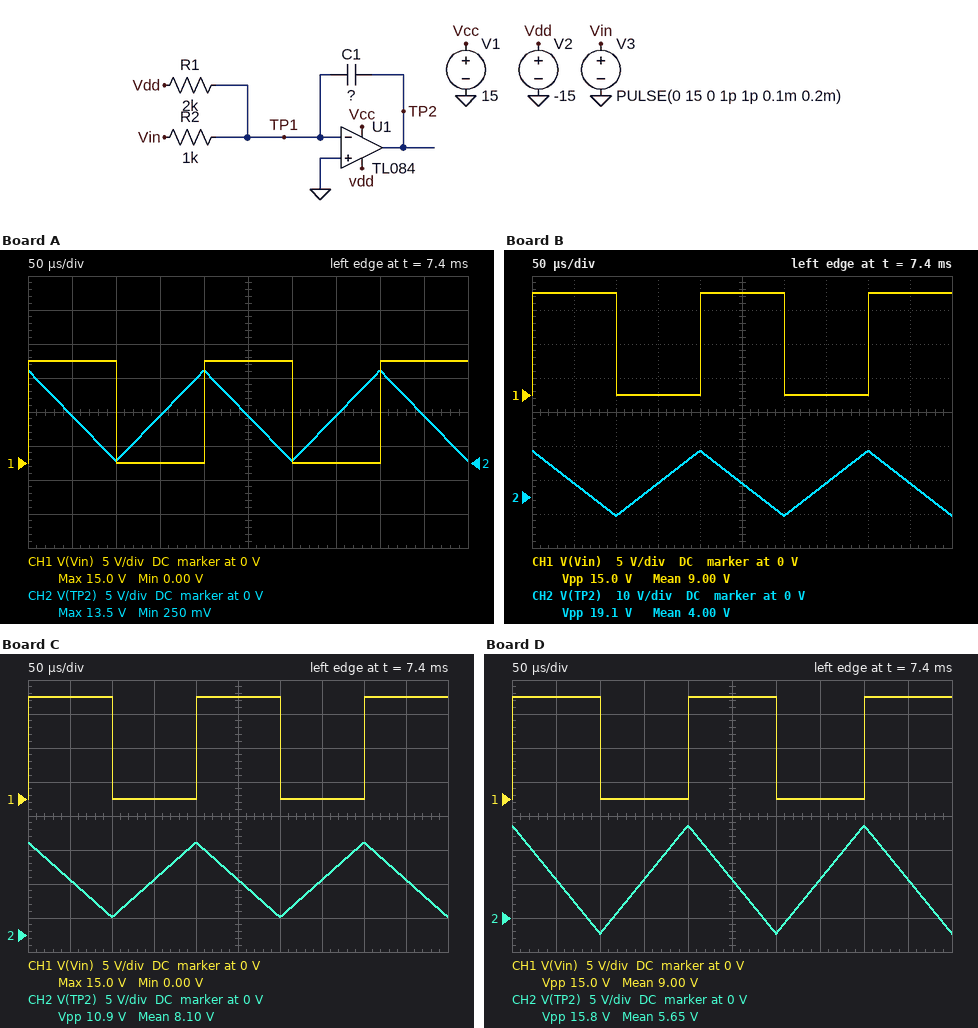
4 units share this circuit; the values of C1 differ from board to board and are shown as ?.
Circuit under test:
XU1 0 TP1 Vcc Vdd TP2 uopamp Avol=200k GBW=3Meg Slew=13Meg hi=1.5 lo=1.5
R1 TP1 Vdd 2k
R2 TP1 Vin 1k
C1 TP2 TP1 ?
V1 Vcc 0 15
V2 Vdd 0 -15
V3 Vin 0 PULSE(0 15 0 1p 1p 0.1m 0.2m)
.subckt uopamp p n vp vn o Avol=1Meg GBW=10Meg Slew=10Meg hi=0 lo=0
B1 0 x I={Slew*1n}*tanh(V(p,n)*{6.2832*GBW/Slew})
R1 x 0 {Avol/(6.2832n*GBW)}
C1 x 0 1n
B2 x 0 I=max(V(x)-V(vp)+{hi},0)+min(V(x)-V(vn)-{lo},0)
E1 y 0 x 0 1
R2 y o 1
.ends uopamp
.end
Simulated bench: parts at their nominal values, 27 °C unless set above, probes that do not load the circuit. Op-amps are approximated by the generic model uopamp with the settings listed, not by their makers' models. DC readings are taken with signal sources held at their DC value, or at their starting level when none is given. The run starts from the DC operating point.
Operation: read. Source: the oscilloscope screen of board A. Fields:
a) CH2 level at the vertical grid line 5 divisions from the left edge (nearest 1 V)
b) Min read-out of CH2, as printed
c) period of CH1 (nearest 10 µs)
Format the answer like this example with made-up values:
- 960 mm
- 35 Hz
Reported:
- 7 V
- 250 mV
- 200 µs
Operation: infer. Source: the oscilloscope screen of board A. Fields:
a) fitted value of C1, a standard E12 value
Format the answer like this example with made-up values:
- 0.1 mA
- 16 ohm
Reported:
- 56 nF
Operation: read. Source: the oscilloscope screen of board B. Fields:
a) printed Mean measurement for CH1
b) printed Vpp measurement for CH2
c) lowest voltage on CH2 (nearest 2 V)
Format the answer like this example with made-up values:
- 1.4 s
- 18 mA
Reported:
- 9.00 V
- 19.1 V
- -6 V
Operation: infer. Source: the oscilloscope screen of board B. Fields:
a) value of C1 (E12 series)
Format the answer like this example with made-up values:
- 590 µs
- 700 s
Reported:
- 39 nF
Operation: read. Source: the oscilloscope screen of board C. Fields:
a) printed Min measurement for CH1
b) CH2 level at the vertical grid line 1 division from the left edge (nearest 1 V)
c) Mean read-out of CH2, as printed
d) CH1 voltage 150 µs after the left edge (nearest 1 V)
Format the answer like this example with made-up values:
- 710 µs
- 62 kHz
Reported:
- 0.00 V
- 8 V
- 8.10 V
- 0 V
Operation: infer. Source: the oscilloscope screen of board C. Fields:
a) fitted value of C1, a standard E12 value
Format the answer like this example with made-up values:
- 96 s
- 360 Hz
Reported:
- 68 nF
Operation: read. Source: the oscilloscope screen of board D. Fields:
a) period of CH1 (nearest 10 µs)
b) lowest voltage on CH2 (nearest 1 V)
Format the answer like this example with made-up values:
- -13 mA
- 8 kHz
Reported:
- 200 µs
- -2 V
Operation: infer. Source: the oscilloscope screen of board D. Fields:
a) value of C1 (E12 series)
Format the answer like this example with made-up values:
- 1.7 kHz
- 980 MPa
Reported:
- 47 nF
